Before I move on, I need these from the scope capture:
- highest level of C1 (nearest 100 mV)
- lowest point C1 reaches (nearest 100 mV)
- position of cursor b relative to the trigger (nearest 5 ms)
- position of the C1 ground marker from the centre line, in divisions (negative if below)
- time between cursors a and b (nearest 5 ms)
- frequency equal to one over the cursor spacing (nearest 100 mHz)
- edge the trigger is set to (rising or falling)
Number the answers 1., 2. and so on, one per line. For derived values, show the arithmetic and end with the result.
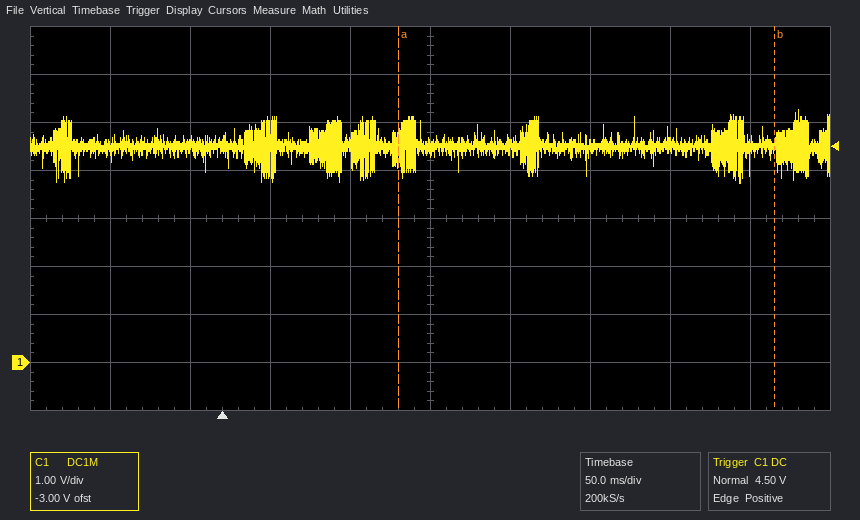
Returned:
1. 5.3 V
2. 3.7 V
3. +345 ms
4. -3.0 div
5. 235 ms
6. 1 / 235 ms ≈ 4.3 Hz
7. rising
